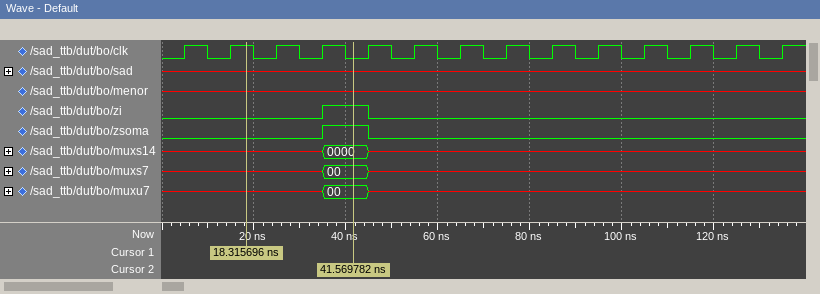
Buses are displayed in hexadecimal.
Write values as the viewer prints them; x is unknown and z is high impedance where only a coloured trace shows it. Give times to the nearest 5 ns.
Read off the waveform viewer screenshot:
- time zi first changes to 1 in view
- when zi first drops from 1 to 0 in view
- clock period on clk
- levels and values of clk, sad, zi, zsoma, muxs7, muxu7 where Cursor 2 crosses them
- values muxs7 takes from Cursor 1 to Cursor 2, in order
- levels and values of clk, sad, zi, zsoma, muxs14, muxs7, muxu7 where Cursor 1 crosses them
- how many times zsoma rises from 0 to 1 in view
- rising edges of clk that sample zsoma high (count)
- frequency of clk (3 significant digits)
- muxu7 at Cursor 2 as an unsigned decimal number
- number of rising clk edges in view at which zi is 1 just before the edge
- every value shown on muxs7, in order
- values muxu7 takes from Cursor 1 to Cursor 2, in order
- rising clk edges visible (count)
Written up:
35 ns
45 ns
10 ns
clk=0, sad=x, zi=1, zsoma=1, muxs7=00, muxu7=00
x, 00
clk=1, sad=x, zi=0, zsoma=0, muxs14=x, muxs7=x, muxu7=x
1
1
100 MHz
0
1
x, 00, x
x, 00
14
